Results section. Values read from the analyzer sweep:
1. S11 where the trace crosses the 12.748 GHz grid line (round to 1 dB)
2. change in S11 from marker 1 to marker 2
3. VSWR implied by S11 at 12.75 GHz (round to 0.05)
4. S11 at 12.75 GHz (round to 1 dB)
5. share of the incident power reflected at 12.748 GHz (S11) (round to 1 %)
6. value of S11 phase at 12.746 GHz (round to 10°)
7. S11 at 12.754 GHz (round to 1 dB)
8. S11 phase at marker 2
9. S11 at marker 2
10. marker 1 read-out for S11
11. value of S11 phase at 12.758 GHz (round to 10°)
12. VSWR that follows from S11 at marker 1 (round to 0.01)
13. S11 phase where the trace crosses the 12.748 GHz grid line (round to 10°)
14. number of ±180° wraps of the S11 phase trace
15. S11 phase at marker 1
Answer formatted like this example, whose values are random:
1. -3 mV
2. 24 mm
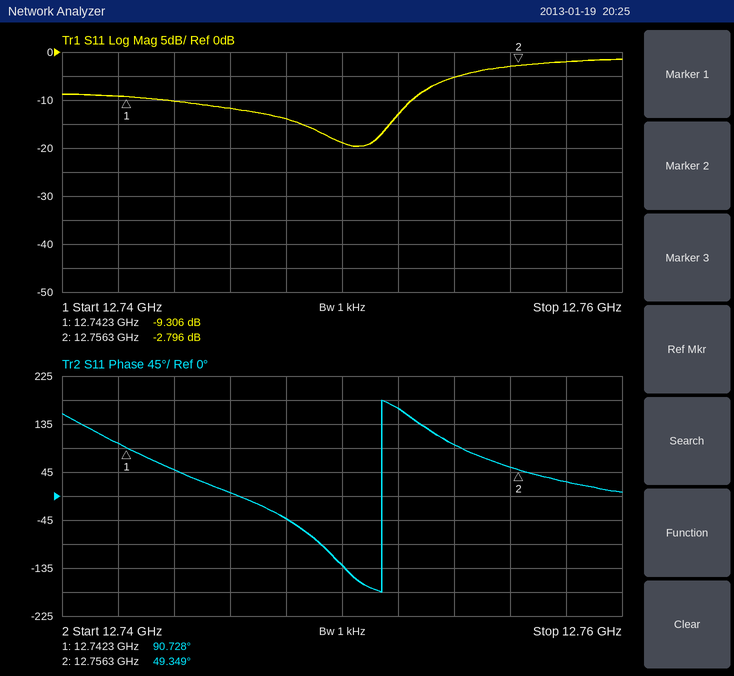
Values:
1. -14 dB
2. 6.510 dB
3. 1.25
4. -19 dB
5. 4 %
6. 10°
7. -5 dB
8. 49.349°
9. -2.796 dB
10. -9.306 dB
11. 30°
12. 2.04
13. -40°
14. 1
15. 90.728°
